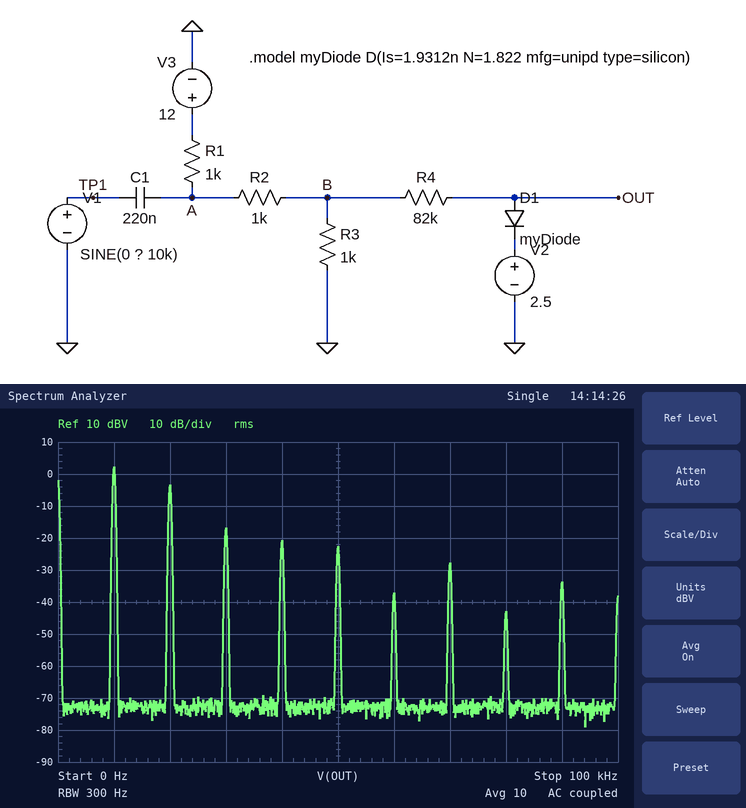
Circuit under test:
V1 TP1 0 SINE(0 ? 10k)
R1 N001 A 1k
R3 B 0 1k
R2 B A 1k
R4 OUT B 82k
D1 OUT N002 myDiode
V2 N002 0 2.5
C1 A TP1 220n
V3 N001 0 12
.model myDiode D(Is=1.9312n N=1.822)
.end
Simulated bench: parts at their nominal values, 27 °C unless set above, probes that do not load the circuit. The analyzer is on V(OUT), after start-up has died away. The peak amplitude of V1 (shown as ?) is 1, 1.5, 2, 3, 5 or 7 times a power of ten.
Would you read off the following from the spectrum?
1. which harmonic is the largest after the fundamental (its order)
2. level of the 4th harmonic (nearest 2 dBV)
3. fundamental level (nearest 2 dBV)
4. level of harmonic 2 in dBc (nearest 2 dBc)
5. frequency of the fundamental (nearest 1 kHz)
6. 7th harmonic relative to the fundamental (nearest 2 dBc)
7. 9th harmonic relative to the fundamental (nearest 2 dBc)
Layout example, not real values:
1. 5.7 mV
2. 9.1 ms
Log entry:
1. 2
2. -20 dBV
3. 2 dBV
4. -6 dBc
5. 10 kHz
6. -30 dBc
7. -36 dBc
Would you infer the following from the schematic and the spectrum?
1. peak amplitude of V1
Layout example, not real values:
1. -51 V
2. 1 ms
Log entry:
1. 10 V
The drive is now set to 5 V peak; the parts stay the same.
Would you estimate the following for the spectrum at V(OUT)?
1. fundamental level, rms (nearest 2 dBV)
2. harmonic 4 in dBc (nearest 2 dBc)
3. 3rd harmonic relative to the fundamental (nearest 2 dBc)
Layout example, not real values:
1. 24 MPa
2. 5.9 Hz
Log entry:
1. -8 dBV
2. -32 dBc
3. -12 dBc
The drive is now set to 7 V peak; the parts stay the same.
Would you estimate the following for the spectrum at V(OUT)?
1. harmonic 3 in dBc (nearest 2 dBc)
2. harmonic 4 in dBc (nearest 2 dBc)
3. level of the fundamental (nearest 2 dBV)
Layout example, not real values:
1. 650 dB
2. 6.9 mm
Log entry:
1. -16 dBc
2. -28 dBc
3. -2 dBV
